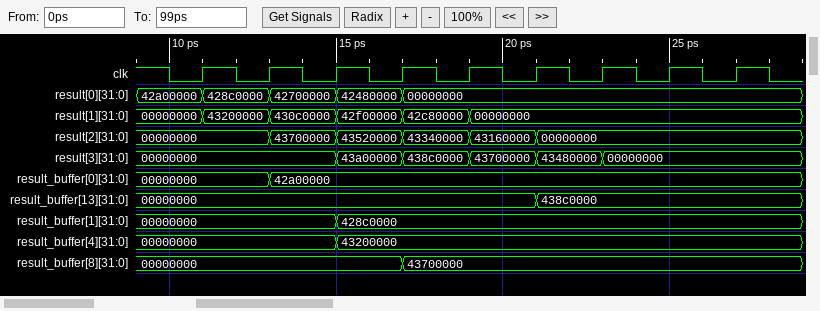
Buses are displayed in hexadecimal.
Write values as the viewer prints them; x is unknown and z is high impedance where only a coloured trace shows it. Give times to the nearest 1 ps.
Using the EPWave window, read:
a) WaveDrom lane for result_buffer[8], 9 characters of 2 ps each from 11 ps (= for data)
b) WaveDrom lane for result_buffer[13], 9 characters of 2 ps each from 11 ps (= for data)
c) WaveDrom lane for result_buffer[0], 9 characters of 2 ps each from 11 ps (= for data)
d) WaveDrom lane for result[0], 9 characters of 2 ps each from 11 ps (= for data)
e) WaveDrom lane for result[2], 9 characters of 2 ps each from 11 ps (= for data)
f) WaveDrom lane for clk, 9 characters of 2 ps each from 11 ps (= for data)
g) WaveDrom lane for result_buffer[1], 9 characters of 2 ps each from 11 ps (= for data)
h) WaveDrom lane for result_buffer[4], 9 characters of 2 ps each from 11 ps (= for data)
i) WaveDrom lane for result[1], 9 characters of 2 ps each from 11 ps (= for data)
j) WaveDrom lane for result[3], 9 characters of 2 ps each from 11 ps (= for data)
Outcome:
{name: 'result_buffer[8]', wave: '=..=.....', data: '00000000 43700000'}
{name: 'result_buffer[13]', wave: '=....=...', data: '00000000 438c0000'}
{name: 'result_buffer[0]', wave: '==.......', data: '00000000 42a00000'}
{name: 'result[0]', wave: '====.....', data: '428c0000 42700000 42480000 00000000'}
{name: 'result[2]', wave: '======...', data: '00000000 43700000 43520000 43340000 43160000 00000000'}
{name: 'clk', wave: 'p........'}
{name: 'result_buffer[1]', wave: '=.=......', data: '00000000 428c0000'}
{name: 'result_buffer[4]', wave: '=.=......', data: '00000000 43200000'}
{name: 'result[1]', wave: '=====....', data: '43200000 430c0000 42f00000 42c80000 00000000'}
{name: 'result[3]', wave: '=.=====..', data: '00000000 43a00000 438c0000 43700000 43480000 00000000'}
